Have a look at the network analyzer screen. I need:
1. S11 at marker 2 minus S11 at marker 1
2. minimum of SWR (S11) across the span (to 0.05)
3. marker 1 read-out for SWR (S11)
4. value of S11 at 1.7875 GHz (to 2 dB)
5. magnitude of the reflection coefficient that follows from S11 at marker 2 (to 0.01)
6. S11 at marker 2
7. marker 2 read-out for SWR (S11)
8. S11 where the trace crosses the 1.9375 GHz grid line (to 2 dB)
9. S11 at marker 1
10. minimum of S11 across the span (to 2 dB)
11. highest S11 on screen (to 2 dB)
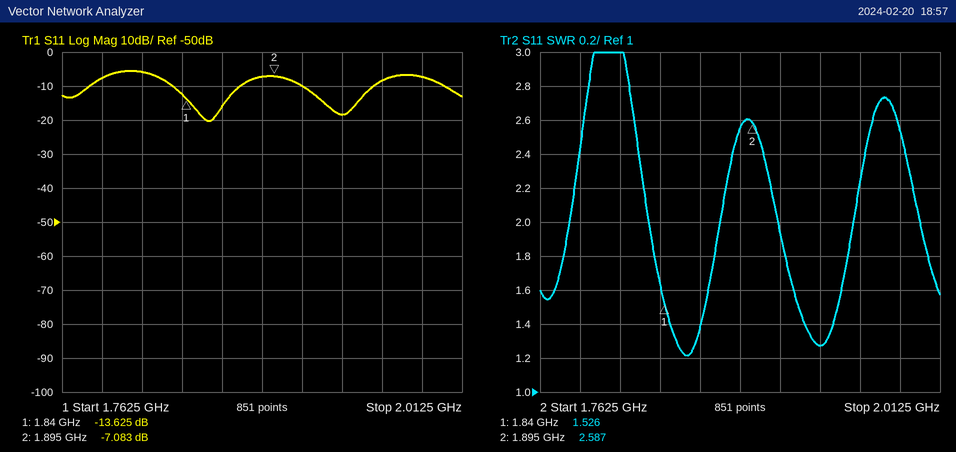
6.542 dB
1.20
1.526
-8 dB
0.44
-7.083 dB
2.587
-18 dB
-13.625 dB
-20 dB
-6 dB
